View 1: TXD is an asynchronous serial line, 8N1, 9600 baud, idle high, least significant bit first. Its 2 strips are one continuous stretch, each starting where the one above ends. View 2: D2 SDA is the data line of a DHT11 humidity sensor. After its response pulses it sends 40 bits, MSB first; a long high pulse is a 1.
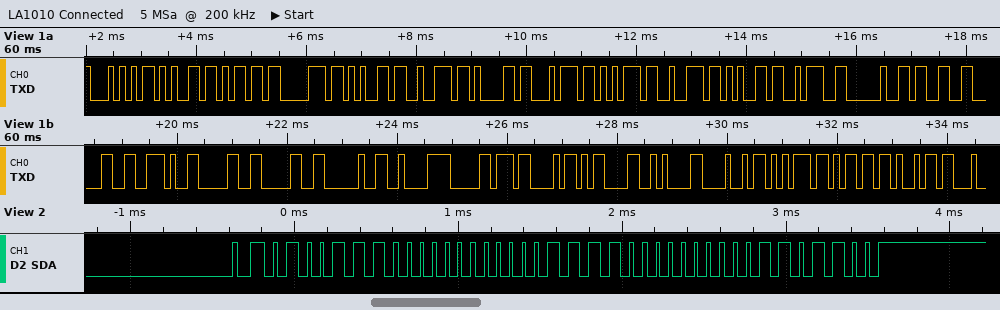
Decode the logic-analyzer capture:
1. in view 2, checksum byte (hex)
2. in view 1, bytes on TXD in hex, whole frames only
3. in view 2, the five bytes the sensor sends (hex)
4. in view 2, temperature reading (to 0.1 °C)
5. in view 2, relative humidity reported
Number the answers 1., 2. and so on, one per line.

1. 0x6C
2. 54 65 6D 70 65 72 61 74 75 72 65 3A 20 33 30 2E 30 30 20 C2 B0 43 0D 0A 48 75 6D 69
3. 4E 00 1E 00 6C
4. 30.0 °C
5. 78 %
